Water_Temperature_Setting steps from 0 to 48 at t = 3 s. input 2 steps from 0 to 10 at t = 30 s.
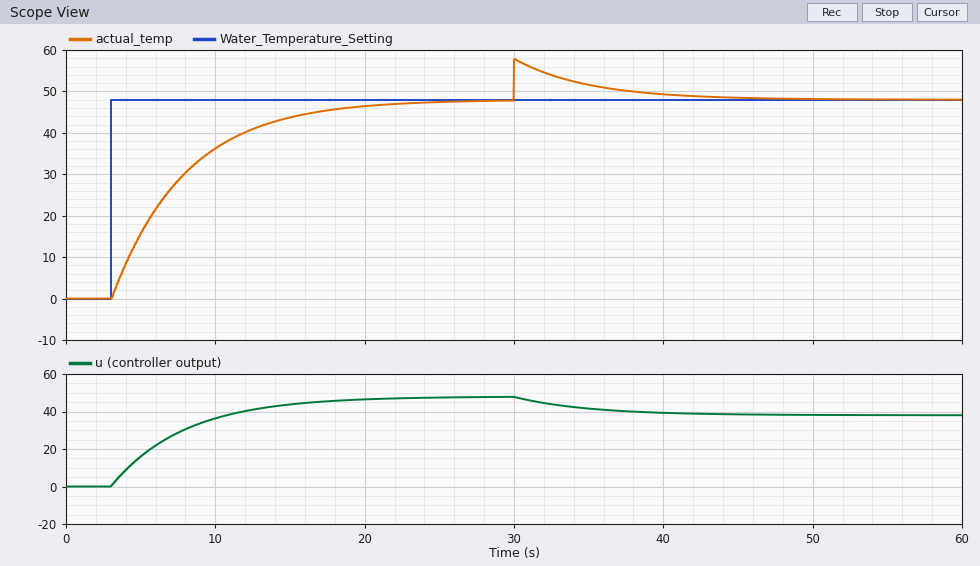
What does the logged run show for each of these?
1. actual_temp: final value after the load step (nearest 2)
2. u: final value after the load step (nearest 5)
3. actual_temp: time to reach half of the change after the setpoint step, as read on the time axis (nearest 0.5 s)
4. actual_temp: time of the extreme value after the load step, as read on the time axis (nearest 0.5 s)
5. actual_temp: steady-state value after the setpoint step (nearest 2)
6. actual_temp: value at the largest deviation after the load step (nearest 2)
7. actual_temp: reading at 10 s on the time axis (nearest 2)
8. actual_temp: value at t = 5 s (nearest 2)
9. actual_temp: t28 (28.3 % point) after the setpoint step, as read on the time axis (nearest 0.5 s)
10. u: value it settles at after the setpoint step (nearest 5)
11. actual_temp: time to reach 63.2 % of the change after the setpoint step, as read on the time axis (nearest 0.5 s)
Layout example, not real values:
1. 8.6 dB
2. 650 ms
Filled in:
1. 48
2. 40
3. 6.5 s
4. 30.0 s
5. 48
6. 58
7. 36
8. 16
9. 4.5 s
10. 50
11. 8.0 s
